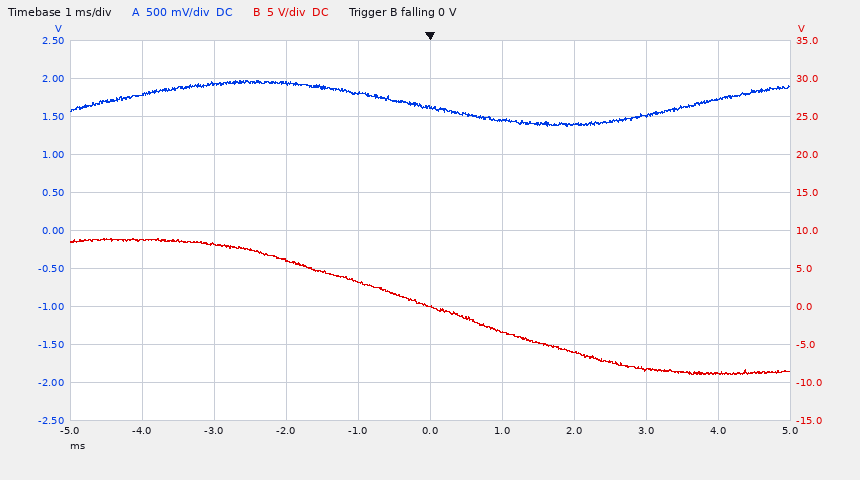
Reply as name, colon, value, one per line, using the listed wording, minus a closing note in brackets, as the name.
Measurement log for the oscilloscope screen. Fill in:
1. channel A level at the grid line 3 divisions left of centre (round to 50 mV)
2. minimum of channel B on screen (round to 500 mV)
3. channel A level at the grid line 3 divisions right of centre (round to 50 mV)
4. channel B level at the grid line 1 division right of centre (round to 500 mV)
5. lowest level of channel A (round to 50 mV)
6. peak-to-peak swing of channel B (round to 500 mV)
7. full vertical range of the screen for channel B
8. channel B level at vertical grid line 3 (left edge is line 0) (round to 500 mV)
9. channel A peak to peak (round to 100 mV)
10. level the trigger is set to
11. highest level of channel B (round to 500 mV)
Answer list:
channel A level at the grid line 3 divisions left of centre: 1.95 V
minimum of channel B on screen: -9.0 V
channel A level at the grid line 3 divisions right of centre: 1.50 V
channel B level at the grid line 1 division right of centre: -3.5 V
lowest level of channel A: 1.35 V
peak-to-peak swing of channel B: 18.0 V
full vertical range of the screen for channel B: 50 V
channel B level at vertical grid line 3 (left edge is line 0): 6.0 V
channel A peak to peak: 600 mV
level the trigger is set to: 0 V
highest level of channel B: 9.0 V
